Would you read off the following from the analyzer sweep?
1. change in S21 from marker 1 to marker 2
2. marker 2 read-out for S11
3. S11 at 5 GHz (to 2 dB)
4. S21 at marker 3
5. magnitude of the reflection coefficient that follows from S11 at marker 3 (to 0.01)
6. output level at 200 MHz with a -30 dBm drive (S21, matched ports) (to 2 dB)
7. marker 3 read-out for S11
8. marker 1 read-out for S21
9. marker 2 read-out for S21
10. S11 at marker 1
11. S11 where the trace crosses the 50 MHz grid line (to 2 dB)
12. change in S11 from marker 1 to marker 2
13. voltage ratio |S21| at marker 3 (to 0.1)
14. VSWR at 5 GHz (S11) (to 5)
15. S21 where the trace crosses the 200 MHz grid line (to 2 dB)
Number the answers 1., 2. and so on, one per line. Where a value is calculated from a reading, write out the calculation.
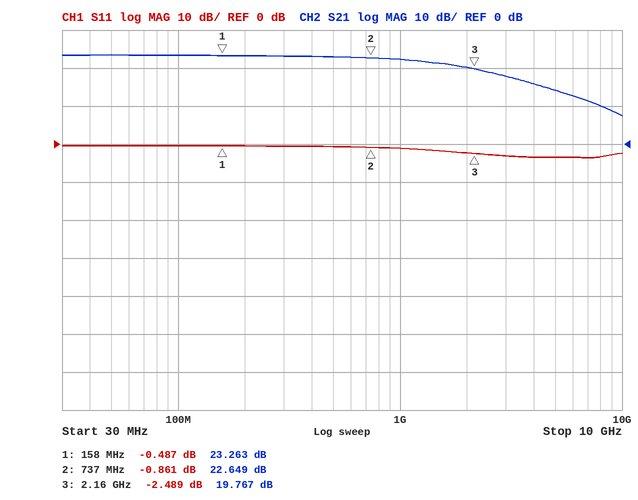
1. 22.649 − (23.263) = -0.614 dB
2. -0.861 dB
3. -4 dB
4. 19.767 dB
5. 10^(-2.489/20) ≈ 0.75
6. -30 dBm + (24 dB) = -6 dBm
7. -2.489 dB
8. 23.263 dB
9. 22.649 dB
10. -0.487 dB
11. 0 dB
12. -0.861 − (-0.487) = -0.374 dB
13. 10^(19.767/20) ≈ 9.7
14. |Γ| = 10^(-4/20) = 0.6310; VSWR = (1 + 0.6310)/(1 − 0.6310) ≈ 4.42, so 5 to the nearest 5
15. 24 dB
